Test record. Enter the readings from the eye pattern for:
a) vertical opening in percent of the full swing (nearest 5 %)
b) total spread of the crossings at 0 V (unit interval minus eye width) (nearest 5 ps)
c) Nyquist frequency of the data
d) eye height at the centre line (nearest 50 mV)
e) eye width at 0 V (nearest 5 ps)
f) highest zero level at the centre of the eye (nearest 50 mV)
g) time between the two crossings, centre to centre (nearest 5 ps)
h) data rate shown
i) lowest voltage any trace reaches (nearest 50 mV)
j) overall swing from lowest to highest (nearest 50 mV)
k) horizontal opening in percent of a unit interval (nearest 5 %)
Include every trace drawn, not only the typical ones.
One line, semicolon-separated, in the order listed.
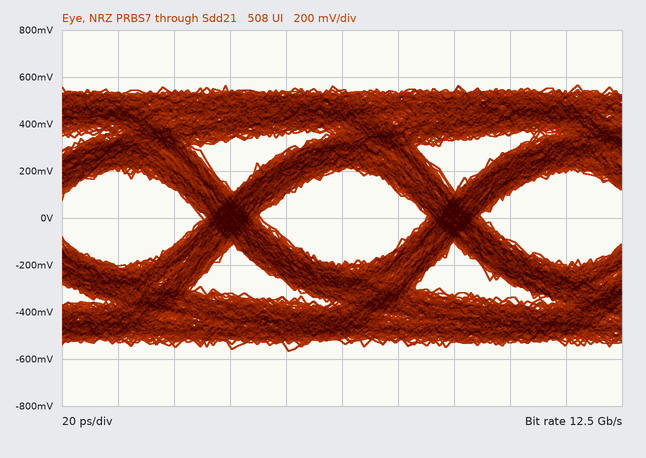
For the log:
35 %; 20 ps; 6.25 GHz; 400 mV; 60 ps; -200 mV; 80 ps; 12.5 Gb/s; -550 mV; 1.15 V; 75 %
